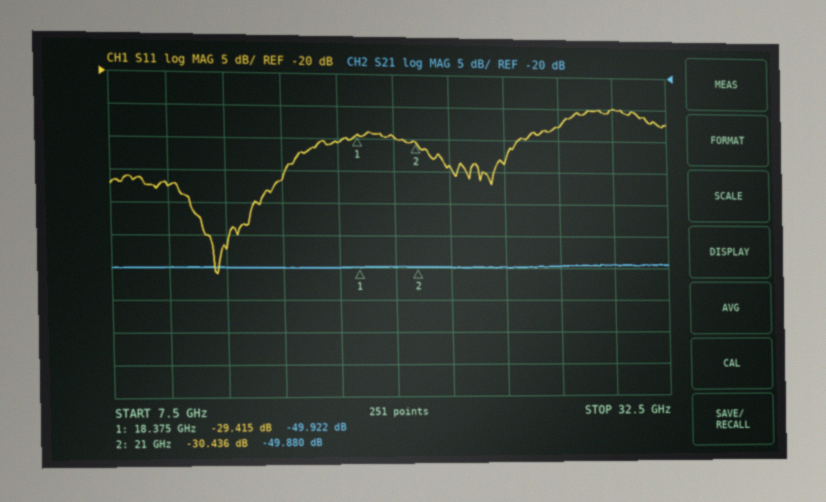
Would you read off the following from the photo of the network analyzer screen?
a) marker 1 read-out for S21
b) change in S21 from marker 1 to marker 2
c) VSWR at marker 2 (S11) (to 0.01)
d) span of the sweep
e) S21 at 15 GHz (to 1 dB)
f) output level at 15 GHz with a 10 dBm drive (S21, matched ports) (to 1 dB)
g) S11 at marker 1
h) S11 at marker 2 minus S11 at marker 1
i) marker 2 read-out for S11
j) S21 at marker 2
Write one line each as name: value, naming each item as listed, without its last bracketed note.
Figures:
marker 1 read-out for S21: -49.922 dB
change in S21 from marker 1 to marker 2: 0.042 dB
VSWR at marker 2 (S11): 1.06
span of the sweep: 25 GHz
S21 at 15 GHz: -50 dB
output level at 15 GHz with a 10 dBm drive (S21, matched ports): -40 dBm
S11 at marker 1: -29.415 dB
S11 at marker 2 minus S11 at marker 1: -1.021 dB
marker 2 read-out for S11: -30.436 dB
S21 at marker 2: -49.880 dB
